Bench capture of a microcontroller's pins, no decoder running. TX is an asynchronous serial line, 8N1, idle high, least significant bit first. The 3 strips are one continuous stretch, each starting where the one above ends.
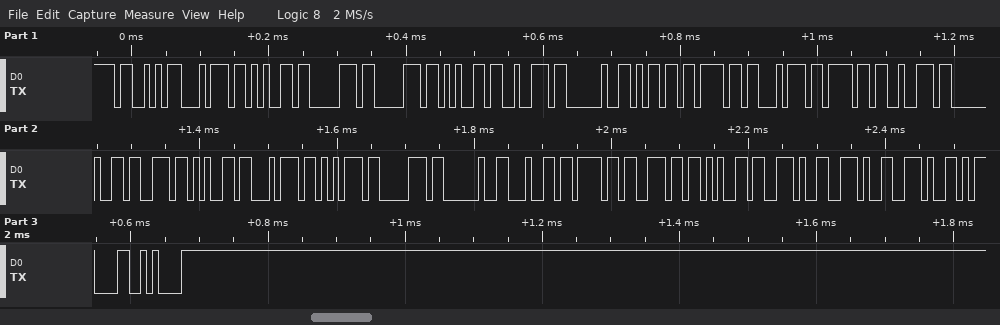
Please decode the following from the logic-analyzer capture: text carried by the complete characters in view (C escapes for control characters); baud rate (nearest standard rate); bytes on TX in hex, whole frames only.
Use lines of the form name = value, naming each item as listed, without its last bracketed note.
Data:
text carried by the complete characters in view = "Stepper motor setup done...\r\n"
baud rate = 115200 baud
bytes on TX in hex, whole frames only = 53 74 65 70 70 65 72 20 6D 6F 74 6F 72 20 73 65 74 75 70 20 64 6F 6E 65 2E 2E 2E 0D 0A
